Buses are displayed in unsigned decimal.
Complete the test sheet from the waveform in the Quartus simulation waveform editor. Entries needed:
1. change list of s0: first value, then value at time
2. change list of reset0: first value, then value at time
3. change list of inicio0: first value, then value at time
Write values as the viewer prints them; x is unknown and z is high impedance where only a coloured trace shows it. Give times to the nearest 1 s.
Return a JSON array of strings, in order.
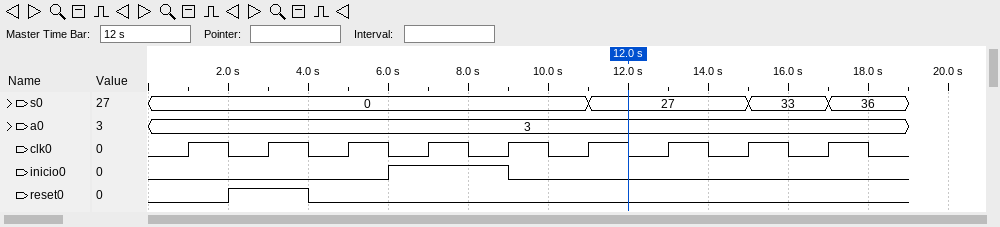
["0, 27 at 11 s, 33 at 15 s, 36 at 17 s", "0, 1 at 2 s, 0 at 4 s", "0, 1 at 6 s, 0 at 9 s"]
